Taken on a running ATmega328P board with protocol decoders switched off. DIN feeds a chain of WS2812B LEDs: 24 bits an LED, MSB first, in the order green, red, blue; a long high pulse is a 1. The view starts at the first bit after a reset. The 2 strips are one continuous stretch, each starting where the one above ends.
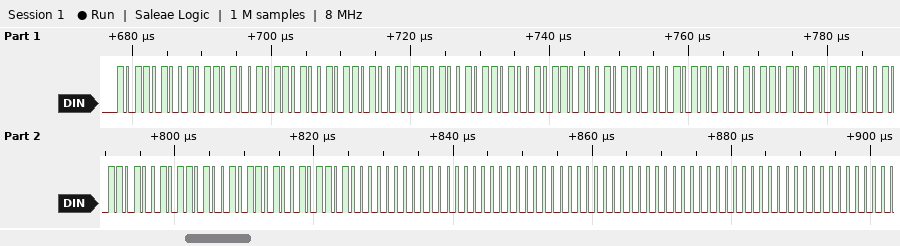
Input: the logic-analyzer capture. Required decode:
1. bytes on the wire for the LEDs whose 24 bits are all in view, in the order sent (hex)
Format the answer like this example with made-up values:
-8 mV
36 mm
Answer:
B4 B4 B4 B4 B4 B4 B4 B4 B4 B4 B4 B4 B4 B4 B4 00 00 00 00 00 00
